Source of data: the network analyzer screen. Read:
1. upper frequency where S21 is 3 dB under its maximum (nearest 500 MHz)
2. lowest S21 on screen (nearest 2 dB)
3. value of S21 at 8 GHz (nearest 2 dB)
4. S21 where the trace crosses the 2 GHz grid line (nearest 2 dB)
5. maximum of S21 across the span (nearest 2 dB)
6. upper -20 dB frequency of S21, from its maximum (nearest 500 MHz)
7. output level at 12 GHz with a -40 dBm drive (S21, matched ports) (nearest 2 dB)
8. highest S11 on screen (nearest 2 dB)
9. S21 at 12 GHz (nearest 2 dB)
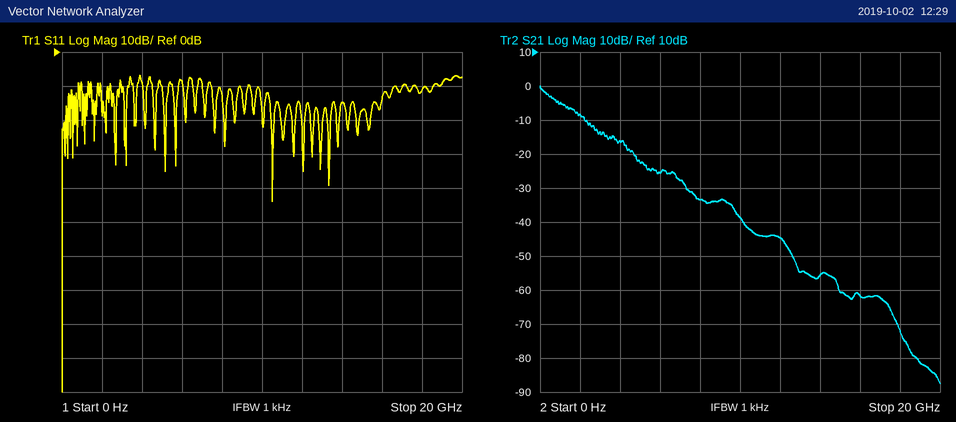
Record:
500 MHz
-88 dB
-34 dB
-8 dB
0 dB
4.5 GHz
-84 dBm
-6 dB
-44 dB
